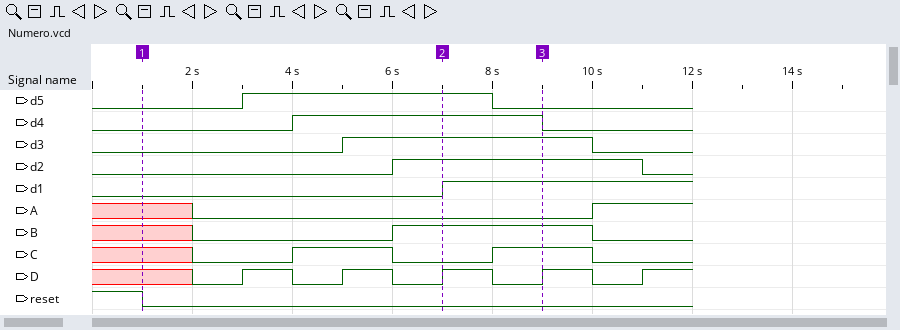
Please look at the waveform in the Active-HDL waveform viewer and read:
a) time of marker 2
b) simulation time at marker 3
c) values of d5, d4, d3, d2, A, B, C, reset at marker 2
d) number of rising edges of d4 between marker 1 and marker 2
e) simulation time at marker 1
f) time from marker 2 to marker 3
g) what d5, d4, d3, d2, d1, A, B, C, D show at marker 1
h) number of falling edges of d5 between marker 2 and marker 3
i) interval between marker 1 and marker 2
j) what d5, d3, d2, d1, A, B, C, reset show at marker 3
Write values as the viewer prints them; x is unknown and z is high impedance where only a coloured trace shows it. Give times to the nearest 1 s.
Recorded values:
7 s
9 s
d5=1, d4=1, d3=1, d2=1, A=0, B=1, C=0, reset=0
1
1 s
2 s
d5=0, d4=0, d3=0, d2=0, d1=0, A=x, B=x, C=x, D=x
1
6 s
d5=0, d3=1, d2=1, d1=1, A=0, B=1, C=1, reset=0
